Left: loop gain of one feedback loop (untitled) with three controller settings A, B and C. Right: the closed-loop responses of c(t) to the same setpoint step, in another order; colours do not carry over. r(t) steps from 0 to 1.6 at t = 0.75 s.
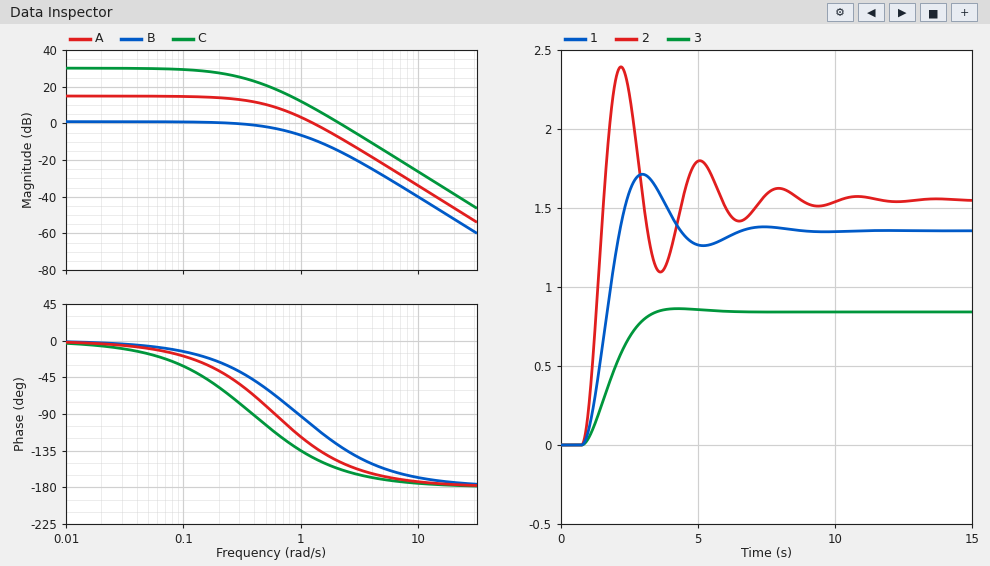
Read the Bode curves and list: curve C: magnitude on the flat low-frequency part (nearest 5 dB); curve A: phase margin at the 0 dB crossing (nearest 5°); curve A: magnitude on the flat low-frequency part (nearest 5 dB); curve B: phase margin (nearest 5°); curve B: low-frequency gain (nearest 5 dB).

30 dB
50°
15 dB
145°
0 dB
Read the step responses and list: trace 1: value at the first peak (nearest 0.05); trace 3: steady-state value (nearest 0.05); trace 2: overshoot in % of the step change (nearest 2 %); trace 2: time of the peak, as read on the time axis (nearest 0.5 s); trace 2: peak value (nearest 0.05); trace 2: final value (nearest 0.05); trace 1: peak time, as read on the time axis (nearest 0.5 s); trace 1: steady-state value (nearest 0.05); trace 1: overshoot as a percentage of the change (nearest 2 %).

1.70
0.85
54 %
2.0 s
2.40
1.55
3.0 s
1.35
26 %
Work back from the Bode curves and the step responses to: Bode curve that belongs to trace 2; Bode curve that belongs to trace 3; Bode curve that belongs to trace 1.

C
B
A
